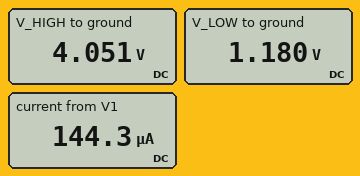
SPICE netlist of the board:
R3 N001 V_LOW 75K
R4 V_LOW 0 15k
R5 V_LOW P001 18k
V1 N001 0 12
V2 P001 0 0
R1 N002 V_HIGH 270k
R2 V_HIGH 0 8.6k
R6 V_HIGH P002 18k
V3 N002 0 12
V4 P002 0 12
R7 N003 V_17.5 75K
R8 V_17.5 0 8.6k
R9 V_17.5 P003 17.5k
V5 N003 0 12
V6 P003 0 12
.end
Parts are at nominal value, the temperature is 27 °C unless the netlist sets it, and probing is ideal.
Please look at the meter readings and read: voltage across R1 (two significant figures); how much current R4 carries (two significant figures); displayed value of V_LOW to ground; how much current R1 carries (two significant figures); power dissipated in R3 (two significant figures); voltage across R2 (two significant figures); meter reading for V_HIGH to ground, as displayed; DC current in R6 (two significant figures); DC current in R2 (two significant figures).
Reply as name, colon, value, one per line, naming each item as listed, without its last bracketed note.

voltage across R1: 7.9 V
how much current R4 carries: 79 µA
displayed value of V_LOW to ground: 1.180 V
how much current R1 carries: 29 µA
power dissipated in R3: 1.6 mW
voltage across R2: 4.1 V
meter reading for V_HIGH to ground, as displayed: 4.051 V
DC current in R6: 440 µA
DC current in R2: 470 µA
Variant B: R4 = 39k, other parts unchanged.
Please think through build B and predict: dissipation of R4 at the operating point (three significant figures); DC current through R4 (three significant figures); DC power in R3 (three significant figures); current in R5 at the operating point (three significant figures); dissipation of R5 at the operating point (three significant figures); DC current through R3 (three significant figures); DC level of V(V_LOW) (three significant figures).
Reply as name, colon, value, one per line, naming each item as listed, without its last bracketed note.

dissipation of R4 at the operating point: 73.5 µW
DC current through R4: 43.4 µA
DC power in R3: 1.42 mW
current in R5 at the operating point: 94.0 µA
dissipation of R5 at the operating point: 159 µW
DC current through R3: 137 µA
DC level of V(V_LOW): 1.69 V
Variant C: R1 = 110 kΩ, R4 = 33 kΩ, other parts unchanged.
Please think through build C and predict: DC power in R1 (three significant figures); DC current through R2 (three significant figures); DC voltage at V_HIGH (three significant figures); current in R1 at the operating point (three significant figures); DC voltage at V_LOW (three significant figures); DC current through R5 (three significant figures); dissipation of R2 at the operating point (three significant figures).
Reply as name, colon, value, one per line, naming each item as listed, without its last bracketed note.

DC power in R1: 541 µW
DC current through R2: 499 µA
DC voltage at V_HIGH: 4.29 V
current in R1 at the operating point: 70.1 µA
DC voltage at V_LOW: 1.61 V
DC current through R5: 89.6 µA
dissipation of R2 at the operating point: 2.14 mW
